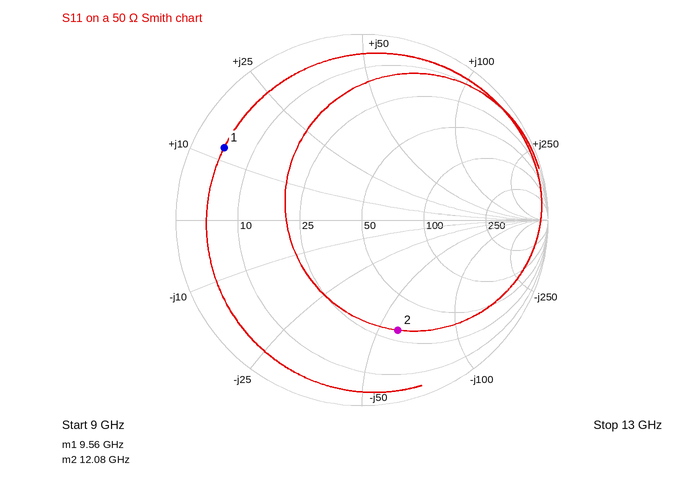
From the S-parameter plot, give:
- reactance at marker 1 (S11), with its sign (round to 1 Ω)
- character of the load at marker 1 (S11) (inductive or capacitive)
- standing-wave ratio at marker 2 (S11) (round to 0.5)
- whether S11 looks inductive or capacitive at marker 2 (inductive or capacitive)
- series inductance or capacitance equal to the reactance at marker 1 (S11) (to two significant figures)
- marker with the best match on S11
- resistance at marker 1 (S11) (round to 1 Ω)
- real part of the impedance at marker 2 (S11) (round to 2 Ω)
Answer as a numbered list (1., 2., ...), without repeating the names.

1. +12 Ω
2. inductive
3. 4.5
4. capacitive
5. 200 pH
6. marker 2
7. 5 Ω
8. 30 Ω
